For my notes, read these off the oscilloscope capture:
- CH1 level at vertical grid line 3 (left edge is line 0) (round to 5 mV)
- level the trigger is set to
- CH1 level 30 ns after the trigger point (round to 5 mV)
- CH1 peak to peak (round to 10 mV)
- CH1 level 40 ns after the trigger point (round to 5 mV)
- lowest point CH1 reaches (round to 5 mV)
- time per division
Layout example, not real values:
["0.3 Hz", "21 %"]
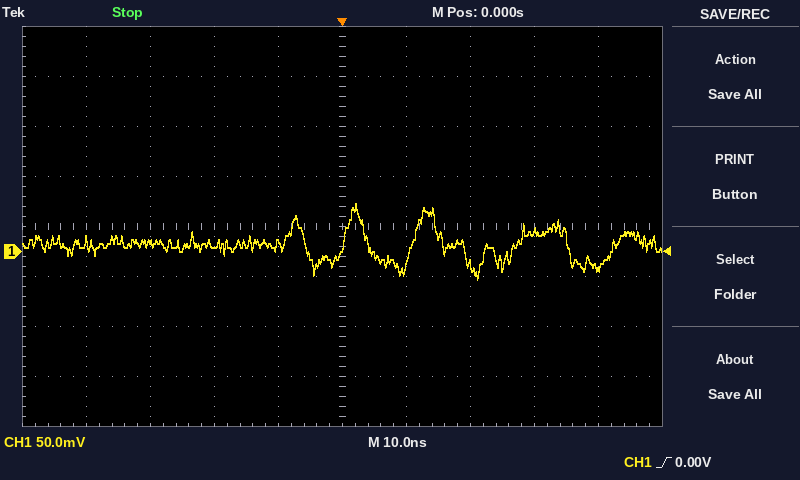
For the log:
["5 mV", "0.00 V", "20 mV", "80 mV", "-15 mV", "-30 mV", "10 ns"]
